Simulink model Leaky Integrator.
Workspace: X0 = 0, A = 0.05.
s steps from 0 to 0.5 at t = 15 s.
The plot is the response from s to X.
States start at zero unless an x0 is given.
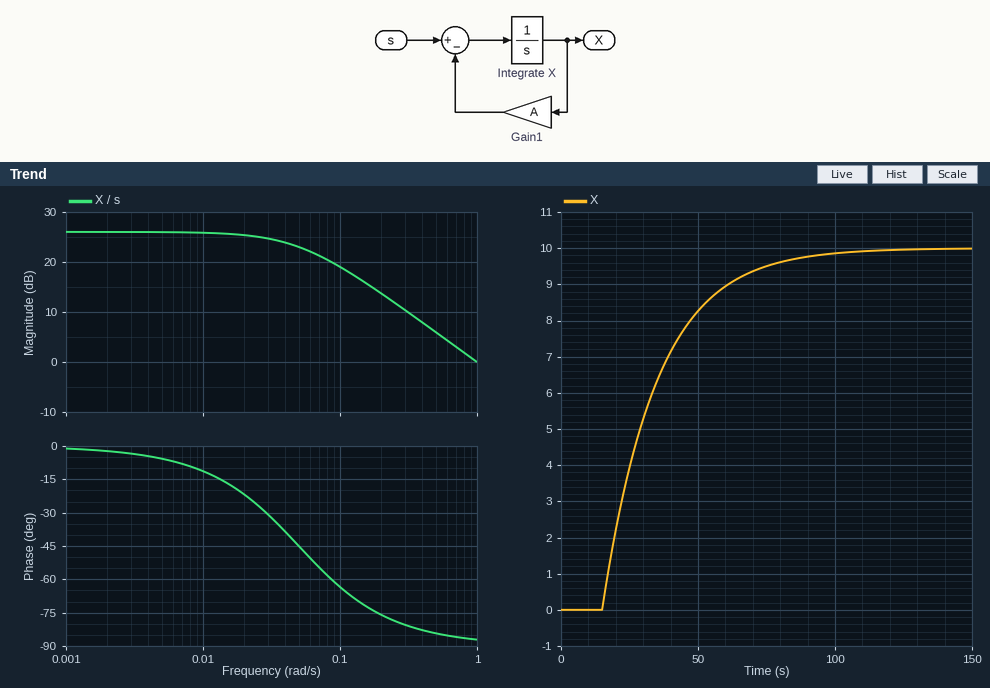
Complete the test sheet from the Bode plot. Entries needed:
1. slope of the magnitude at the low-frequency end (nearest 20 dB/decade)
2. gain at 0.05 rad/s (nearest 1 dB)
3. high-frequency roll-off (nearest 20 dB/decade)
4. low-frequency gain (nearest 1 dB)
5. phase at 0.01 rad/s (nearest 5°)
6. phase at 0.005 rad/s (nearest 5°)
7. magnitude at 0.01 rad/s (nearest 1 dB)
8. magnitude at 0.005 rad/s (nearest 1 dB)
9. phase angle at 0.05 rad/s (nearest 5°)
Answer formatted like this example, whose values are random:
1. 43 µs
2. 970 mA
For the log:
1. 0 dB/decade
2. 23 dB
3. -20 dB/decade
4. 26 dB
5. -10°
6. -5°
7. 26 dB
8. 26 dB
9. -45°
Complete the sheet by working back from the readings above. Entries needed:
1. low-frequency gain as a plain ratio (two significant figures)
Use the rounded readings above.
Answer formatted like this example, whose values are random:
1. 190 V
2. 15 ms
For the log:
1. 20
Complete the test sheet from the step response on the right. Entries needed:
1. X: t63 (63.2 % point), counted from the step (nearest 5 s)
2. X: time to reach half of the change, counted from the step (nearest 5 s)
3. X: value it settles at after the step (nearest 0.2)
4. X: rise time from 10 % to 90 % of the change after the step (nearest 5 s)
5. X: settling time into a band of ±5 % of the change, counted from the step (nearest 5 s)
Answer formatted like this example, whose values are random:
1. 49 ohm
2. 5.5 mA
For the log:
1. 20 s
2. 15 s
3. 10.0
4. 45 s
5. 60 s
